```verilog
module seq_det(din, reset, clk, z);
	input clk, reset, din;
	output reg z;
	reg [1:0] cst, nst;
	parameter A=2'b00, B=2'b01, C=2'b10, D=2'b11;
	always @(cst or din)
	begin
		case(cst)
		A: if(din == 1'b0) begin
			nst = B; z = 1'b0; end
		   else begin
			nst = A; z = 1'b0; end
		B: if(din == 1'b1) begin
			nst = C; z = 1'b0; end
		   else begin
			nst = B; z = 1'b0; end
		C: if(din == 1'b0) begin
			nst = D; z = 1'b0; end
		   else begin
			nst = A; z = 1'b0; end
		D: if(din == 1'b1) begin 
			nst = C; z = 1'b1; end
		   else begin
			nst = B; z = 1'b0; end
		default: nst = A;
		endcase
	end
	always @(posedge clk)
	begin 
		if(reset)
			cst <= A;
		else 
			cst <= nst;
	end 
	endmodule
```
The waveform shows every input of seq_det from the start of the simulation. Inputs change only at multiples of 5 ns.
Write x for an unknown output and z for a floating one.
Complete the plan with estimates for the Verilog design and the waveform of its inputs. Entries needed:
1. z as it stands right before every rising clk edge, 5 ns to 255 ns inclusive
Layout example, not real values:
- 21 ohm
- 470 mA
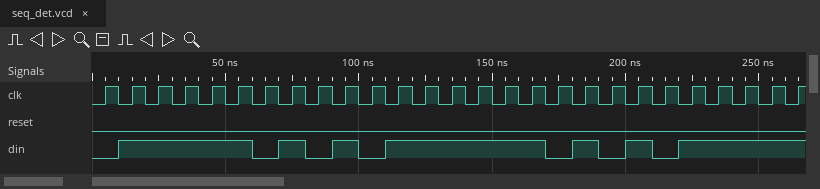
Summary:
- x 0 0 0 0 0 0 0 0 1 0 1 0 0 0 0 0 0 0 0 1 0 1 0 0 0
